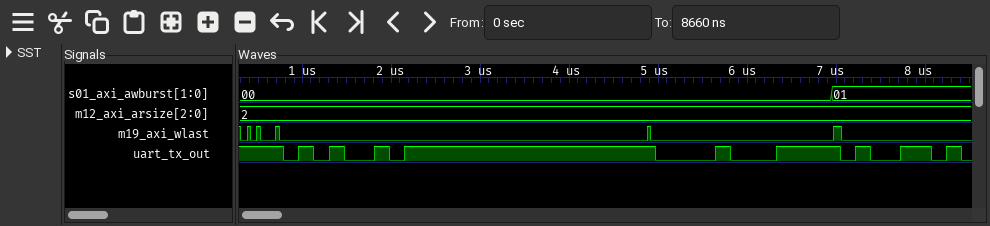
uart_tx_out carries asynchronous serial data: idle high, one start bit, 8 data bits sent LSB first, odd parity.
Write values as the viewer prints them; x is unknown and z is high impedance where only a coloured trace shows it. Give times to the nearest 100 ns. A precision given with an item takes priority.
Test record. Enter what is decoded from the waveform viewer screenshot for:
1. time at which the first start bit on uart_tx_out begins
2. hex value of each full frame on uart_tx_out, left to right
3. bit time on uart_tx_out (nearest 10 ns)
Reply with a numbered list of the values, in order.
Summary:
1. 800 ns
2. A5, 88
3. 170 ns
